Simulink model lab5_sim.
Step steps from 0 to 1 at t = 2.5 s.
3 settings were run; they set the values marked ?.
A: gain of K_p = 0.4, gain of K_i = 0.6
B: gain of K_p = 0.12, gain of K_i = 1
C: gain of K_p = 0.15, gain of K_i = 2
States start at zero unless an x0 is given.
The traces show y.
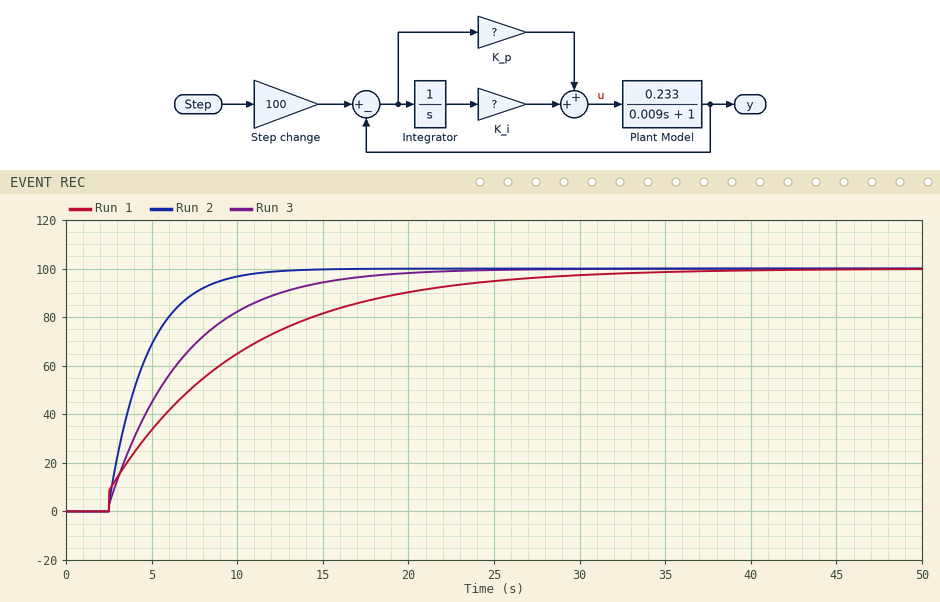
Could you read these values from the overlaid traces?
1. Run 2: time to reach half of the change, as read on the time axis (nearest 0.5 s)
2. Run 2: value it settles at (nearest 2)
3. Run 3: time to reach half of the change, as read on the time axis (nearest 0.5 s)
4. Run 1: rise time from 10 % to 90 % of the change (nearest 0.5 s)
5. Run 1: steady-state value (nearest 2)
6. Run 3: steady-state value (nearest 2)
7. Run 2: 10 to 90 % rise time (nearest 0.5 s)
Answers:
4.0 s
100
5.5 s
17.0 s
100
100
5.0 s
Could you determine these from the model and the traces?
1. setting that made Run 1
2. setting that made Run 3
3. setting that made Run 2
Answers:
A
B
C
